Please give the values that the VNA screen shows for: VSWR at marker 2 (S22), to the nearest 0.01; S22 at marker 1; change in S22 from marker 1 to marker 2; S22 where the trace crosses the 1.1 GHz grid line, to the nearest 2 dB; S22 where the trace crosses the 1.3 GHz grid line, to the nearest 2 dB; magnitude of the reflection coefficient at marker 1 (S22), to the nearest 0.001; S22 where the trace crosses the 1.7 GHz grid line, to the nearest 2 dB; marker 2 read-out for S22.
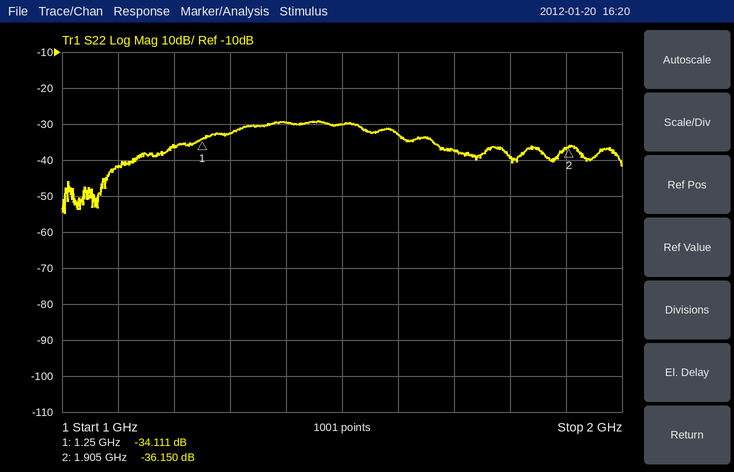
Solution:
1.03
-34.111 dB
-2.039 dB
-42 dB
-32 dB
0.020
-38 dB
-36.150 dB
